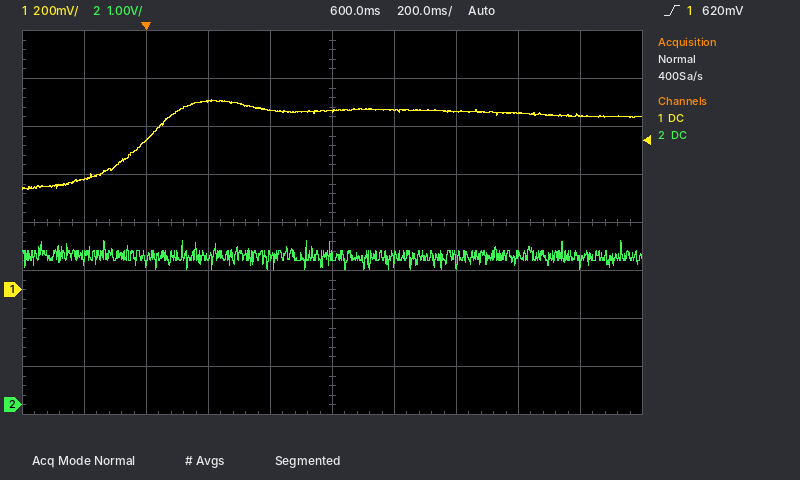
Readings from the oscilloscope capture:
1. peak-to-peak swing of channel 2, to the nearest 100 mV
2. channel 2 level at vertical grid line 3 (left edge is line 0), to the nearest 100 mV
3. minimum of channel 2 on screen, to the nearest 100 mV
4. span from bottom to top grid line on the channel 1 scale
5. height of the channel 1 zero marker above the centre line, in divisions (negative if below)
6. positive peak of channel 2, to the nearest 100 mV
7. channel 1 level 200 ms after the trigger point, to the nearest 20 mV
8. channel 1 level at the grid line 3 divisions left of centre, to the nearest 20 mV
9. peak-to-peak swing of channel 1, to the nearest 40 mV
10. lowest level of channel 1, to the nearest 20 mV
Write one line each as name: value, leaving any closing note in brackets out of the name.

peak-to-peak swing of channel 2, to the nearest 100 mV: 600 mV
channel 2 level at vertical grid line 3 (left edge is line 0), to the nearest 100 mV: 3.1 V
minimum of channel 2 on screen, to the nearest 100 mV: 2.8 V
span from bottom to top grid line on the channel 1 scale: 1.6 V
height of the channel 1 zero marker above the centre line, in divisions: -1.4 div
positive peak of channel 2, to the nearest 100 mV: 3.4 V
channel 1 level 200 ms after the trigger point, to the nearest 20 mV: 780 mV
channel 1 level at the grid line 3 divisions left of centre, to the nearest 20 mV: 620 mV
peak-to-peak swing of channel 1, to the nearest 40 mV: 360 mV
lowest level of channel 1, to the nearest 20 mV: 420 mV
